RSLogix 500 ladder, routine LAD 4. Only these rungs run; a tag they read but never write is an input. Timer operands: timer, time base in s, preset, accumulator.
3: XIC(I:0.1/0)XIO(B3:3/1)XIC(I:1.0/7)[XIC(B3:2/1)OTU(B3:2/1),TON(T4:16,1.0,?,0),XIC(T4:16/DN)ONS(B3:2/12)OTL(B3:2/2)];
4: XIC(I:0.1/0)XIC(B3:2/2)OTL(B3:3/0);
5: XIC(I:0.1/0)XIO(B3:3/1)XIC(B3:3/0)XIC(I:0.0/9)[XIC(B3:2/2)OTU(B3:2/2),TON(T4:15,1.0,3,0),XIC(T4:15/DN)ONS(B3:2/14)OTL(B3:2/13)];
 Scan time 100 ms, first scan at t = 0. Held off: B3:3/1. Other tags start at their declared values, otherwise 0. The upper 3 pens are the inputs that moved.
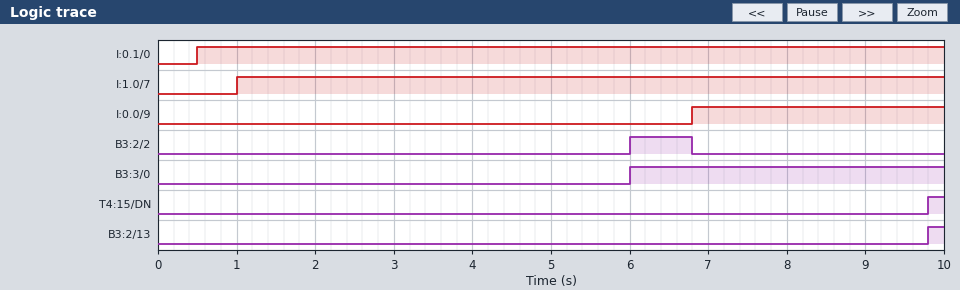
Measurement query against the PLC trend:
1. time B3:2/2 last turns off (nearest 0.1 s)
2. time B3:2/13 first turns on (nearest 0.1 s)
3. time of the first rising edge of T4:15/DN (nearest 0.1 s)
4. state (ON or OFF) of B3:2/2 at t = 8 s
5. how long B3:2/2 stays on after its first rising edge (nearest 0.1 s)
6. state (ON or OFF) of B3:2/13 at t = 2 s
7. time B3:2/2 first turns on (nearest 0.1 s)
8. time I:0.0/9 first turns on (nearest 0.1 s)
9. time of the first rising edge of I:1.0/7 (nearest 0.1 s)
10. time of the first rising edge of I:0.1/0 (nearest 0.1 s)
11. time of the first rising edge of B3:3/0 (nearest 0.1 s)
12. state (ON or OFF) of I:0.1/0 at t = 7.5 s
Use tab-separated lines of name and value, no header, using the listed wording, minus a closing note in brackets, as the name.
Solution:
time B3:2/2 last turns off	6.8 s
time B3:2/13 first turns on	9.8 s
time of the first rising edge of T4:15/DN	9.8 s
state (ON or OFF) of B3:2/2 at t = 8 s	OFF
how long B3:2/2 stays on after its first rising edge	0.8 s
state (ON or OFF) of B3:2/13 at t = 2 s	OFF
time B3:2/2 first turns on	6.0 s
time I:0.0/9 first turns on	6.8 s
time of the first rising edge of I:1.0/7	1.0 s
time of the first rising edge of I:0.1/0	0.5 s
time of the first rising edge of B3:3/0	6.0 s
state (ON or OFF) of I:0.1/0 at t = 7.5 s	ON
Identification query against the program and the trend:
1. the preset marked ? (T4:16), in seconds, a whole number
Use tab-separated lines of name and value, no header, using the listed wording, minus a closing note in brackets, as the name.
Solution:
the preset marked ? (T4:16), in seconds, a whole number	5 s
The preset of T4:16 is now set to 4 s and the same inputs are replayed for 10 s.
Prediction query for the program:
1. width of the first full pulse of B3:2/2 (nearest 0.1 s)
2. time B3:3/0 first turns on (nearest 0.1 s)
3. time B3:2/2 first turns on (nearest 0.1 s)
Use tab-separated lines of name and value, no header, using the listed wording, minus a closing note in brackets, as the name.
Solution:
width of the first full pulse of B3:2/2	1.8 s
time B3:3/0 first turns on	5.0 s
time B3:2/2 first turns on	5.0 s
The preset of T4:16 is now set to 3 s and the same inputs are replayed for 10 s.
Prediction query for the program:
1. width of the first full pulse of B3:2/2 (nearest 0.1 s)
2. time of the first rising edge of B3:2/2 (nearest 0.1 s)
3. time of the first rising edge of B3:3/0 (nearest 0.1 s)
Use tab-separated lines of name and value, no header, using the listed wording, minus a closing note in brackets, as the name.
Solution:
width of the first full pulse of B3:2/2	2.8 s
time of the first rising edge of B3:2/2	4.0 s
time of the first rising edge of B3:3/0	4.0 s
